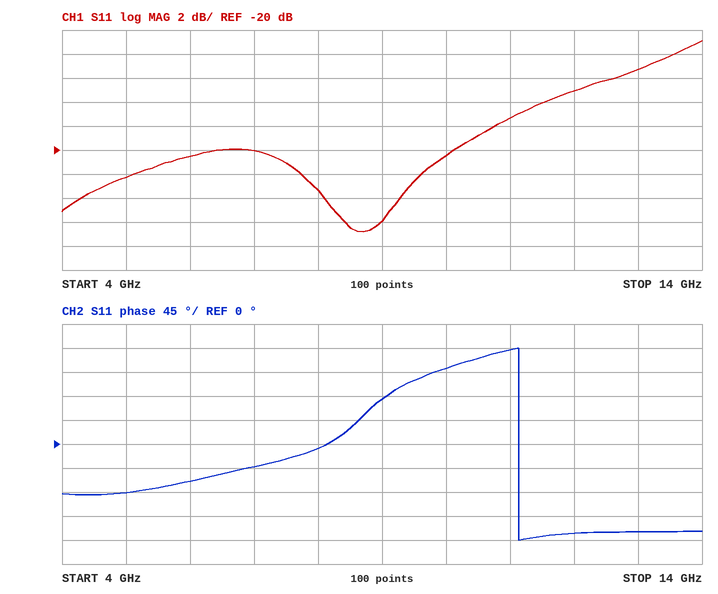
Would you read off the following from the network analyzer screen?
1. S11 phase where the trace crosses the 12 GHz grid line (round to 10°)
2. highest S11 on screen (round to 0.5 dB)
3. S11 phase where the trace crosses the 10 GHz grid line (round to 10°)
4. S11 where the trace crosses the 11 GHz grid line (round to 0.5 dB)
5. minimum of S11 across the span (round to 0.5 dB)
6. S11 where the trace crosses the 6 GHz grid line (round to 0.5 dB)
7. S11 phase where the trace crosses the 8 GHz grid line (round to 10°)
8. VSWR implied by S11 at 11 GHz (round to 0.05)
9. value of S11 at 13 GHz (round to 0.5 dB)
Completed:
-170°
-11.0 dB
140°
-17.5 dB
-27.0 dB
-20.5 dB
-10°
1.30
-13.5 dB
